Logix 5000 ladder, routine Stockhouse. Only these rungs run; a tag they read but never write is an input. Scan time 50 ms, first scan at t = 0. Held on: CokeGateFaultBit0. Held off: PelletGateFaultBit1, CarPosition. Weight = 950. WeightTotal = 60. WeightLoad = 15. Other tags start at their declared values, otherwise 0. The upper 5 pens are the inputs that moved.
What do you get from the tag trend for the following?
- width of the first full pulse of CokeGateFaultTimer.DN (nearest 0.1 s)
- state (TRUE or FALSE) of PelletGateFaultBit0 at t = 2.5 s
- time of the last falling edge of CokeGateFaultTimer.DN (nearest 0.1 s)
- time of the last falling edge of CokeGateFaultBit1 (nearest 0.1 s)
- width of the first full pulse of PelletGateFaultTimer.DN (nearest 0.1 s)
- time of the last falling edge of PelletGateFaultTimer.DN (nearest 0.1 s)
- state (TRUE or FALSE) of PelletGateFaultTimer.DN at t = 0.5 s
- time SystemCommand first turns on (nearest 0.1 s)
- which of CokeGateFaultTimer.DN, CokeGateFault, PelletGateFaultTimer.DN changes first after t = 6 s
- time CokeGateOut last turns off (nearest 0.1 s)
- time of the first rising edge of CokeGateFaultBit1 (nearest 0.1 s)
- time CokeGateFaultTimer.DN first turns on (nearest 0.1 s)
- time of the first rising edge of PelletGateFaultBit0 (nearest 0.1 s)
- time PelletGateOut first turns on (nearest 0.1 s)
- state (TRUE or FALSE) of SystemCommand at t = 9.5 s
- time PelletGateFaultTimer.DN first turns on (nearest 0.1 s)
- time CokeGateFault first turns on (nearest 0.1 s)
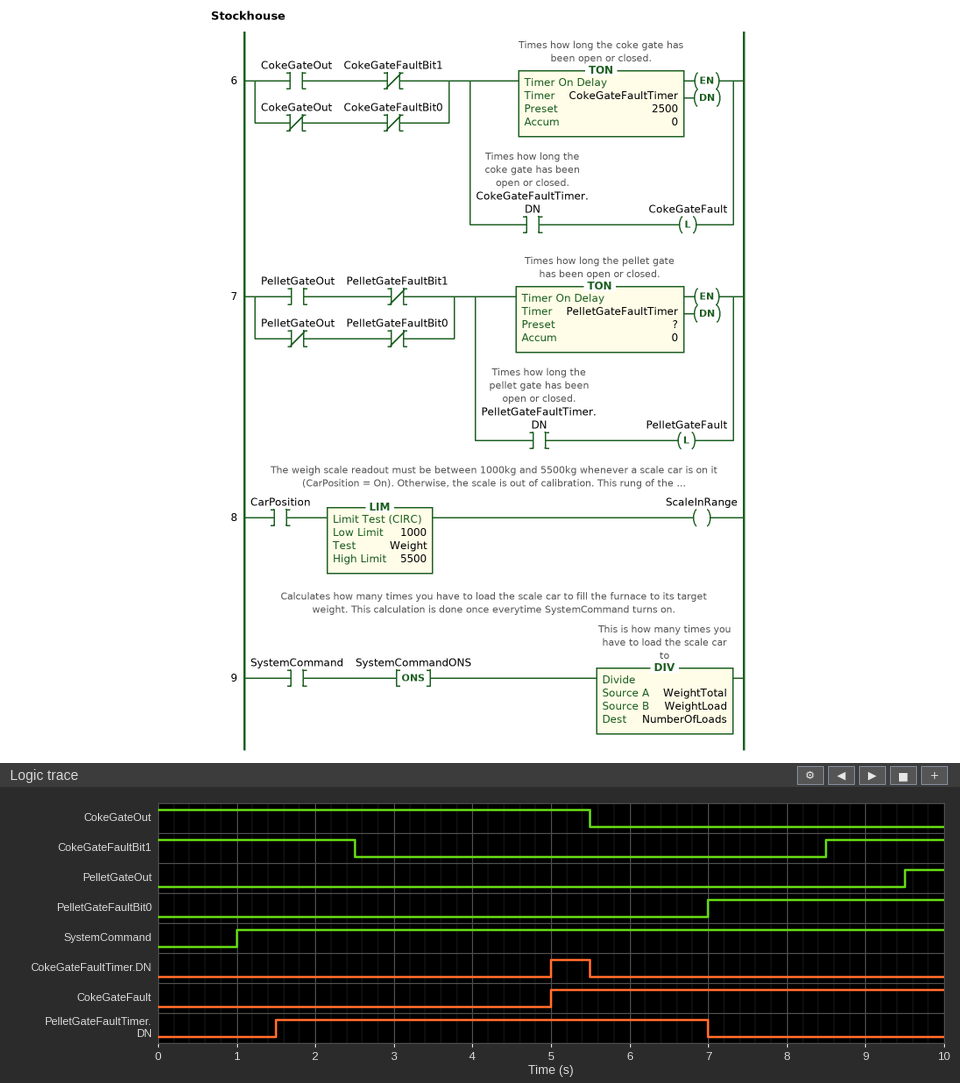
0.5 s
FALSE
5.5 s
2.5 s
5.5 s
7.0 s
FALSE
1.0 s
PelletGateFaultTimer.DN
5.5 s
8.5 s
5.0 s
7.0 s
9.5 s
TRUE
1.5 s
5.0 s
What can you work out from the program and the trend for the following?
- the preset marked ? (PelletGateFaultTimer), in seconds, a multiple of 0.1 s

1.5 s
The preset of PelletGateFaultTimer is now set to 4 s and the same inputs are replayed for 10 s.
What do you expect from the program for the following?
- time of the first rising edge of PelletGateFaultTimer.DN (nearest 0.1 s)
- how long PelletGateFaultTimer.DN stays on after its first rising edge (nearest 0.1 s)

4.0 s
3.0 s
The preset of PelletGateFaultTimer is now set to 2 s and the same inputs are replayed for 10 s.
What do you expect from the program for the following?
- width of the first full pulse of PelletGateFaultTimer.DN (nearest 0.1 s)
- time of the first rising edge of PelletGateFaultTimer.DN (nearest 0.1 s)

5.0 s
2.0 s
